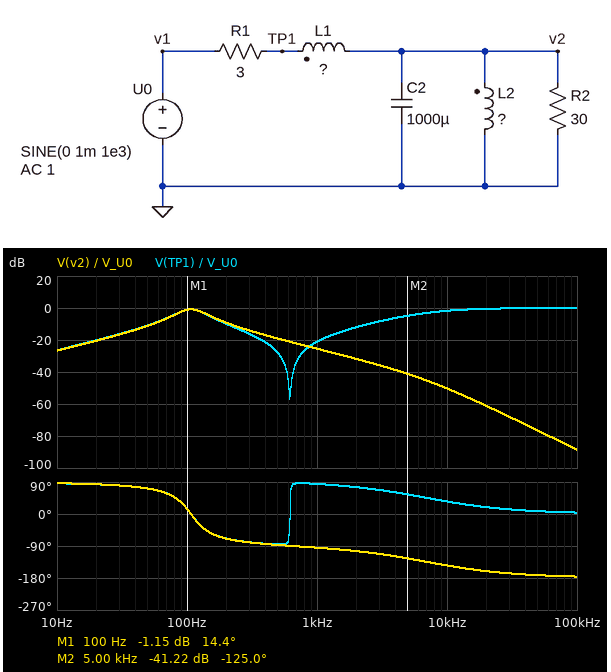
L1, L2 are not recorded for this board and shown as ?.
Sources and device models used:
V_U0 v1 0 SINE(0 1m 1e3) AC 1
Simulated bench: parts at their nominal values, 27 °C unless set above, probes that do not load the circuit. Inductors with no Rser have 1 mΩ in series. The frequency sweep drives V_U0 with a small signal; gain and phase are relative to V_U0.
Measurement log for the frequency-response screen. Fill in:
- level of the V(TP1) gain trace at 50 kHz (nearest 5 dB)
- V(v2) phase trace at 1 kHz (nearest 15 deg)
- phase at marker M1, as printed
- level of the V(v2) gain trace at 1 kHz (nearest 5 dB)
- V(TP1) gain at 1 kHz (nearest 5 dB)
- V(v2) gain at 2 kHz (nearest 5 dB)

0 dB
-90 deg
14.4 deg
-25 dB
-20 dB
-30 dB
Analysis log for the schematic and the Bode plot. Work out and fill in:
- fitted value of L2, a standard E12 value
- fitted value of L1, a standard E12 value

2.2 mH
68 µH
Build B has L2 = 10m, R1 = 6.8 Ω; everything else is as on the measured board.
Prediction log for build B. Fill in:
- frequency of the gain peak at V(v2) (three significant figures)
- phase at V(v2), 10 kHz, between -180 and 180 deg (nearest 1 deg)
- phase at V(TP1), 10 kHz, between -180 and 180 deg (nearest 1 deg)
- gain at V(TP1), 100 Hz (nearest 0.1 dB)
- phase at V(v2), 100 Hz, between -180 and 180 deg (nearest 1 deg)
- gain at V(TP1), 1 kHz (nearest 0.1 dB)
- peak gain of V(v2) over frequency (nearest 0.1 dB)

50.4 Hz
-122 deg
58 deg
-10.8 dB
-69 deg
-28.1 dB
-1.8 dB
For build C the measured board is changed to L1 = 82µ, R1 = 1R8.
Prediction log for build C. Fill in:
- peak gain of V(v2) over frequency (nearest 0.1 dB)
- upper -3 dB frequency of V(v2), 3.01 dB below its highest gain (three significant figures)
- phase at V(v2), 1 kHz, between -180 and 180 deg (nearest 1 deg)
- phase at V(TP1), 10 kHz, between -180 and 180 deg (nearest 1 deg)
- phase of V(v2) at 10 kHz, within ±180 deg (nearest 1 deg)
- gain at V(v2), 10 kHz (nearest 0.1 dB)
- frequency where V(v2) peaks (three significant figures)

-0.5 dB
167 Hz
-101 deg
19 deg
-161 deg
-50.7 dB
109 Hz
